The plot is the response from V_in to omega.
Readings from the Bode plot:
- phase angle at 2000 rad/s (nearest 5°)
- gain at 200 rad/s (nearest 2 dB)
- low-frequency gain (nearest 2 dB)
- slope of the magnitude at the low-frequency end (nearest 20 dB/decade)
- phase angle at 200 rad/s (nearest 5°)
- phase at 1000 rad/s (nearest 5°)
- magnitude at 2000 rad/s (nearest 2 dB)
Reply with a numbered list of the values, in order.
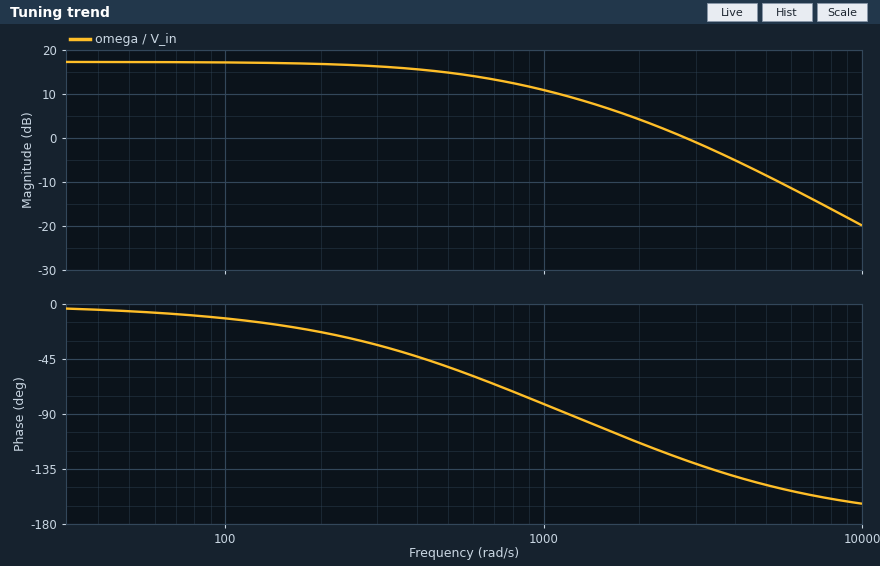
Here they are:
1. -115°
2. 16 dB
3. 18 dB
4. 0 dB/decade
5. -25°
6. -80°
7. 4 dB
